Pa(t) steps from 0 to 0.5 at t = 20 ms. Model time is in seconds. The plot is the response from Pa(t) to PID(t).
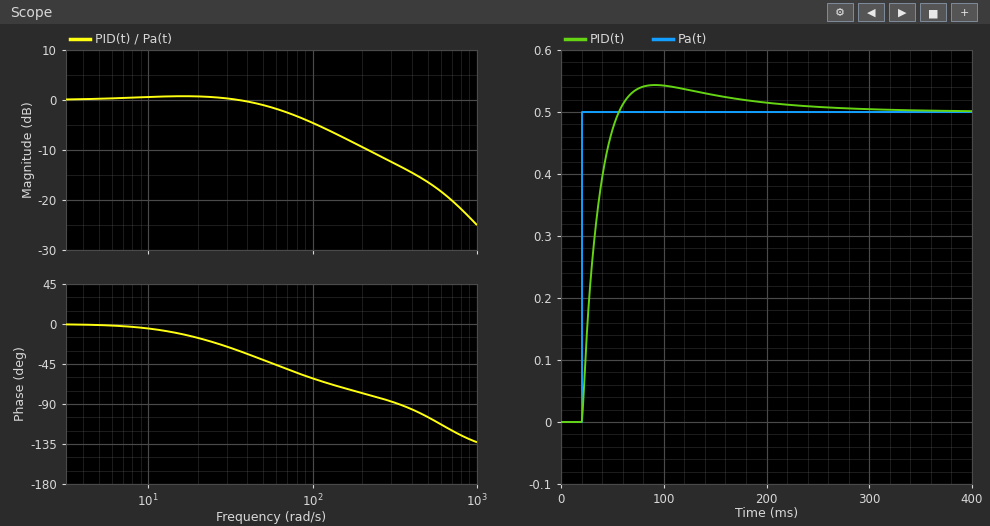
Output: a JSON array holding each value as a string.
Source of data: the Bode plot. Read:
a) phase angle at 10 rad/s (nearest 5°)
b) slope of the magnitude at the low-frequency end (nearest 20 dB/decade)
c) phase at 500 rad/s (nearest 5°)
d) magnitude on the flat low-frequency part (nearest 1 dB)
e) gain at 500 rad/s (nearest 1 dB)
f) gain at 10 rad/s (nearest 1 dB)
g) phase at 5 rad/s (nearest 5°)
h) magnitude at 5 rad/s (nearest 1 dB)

["-5°", "0 dB/decade", "-105°", "0 dB", "-16 dB", "1 dB", "0°", "0 dB"]
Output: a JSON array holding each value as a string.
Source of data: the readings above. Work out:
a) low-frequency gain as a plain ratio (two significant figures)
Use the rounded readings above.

["1.0"]
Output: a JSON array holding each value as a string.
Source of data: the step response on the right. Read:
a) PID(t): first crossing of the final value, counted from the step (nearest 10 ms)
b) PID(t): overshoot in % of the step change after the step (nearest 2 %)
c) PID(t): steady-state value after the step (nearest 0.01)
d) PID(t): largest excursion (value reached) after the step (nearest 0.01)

["40 ms", "8 %", "0.50", "0.54"]
